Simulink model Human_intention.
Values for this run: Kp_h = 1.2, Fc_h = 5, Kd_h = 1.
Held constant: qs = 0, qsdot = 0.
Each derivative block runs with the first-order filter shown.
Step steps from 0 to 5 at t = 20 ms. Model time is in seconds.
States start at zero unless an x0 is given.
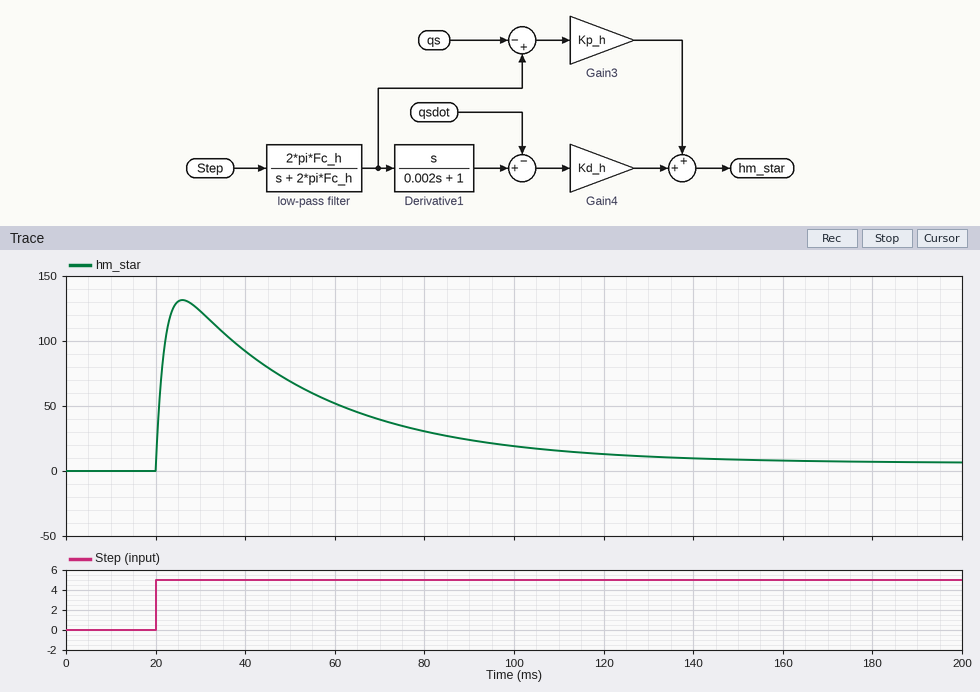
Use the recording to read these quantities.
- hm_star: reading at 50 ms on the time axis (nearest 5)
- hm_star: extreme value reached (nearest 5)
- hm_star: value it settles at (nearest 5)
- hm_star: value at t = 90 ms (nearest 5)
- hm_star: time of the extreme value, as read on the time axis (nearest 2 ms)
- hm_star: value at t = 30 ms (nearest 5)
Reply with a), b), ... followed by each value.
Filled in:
a) 70
b) 130
c) 5
d) 25
e) 26 ms
f) 125
